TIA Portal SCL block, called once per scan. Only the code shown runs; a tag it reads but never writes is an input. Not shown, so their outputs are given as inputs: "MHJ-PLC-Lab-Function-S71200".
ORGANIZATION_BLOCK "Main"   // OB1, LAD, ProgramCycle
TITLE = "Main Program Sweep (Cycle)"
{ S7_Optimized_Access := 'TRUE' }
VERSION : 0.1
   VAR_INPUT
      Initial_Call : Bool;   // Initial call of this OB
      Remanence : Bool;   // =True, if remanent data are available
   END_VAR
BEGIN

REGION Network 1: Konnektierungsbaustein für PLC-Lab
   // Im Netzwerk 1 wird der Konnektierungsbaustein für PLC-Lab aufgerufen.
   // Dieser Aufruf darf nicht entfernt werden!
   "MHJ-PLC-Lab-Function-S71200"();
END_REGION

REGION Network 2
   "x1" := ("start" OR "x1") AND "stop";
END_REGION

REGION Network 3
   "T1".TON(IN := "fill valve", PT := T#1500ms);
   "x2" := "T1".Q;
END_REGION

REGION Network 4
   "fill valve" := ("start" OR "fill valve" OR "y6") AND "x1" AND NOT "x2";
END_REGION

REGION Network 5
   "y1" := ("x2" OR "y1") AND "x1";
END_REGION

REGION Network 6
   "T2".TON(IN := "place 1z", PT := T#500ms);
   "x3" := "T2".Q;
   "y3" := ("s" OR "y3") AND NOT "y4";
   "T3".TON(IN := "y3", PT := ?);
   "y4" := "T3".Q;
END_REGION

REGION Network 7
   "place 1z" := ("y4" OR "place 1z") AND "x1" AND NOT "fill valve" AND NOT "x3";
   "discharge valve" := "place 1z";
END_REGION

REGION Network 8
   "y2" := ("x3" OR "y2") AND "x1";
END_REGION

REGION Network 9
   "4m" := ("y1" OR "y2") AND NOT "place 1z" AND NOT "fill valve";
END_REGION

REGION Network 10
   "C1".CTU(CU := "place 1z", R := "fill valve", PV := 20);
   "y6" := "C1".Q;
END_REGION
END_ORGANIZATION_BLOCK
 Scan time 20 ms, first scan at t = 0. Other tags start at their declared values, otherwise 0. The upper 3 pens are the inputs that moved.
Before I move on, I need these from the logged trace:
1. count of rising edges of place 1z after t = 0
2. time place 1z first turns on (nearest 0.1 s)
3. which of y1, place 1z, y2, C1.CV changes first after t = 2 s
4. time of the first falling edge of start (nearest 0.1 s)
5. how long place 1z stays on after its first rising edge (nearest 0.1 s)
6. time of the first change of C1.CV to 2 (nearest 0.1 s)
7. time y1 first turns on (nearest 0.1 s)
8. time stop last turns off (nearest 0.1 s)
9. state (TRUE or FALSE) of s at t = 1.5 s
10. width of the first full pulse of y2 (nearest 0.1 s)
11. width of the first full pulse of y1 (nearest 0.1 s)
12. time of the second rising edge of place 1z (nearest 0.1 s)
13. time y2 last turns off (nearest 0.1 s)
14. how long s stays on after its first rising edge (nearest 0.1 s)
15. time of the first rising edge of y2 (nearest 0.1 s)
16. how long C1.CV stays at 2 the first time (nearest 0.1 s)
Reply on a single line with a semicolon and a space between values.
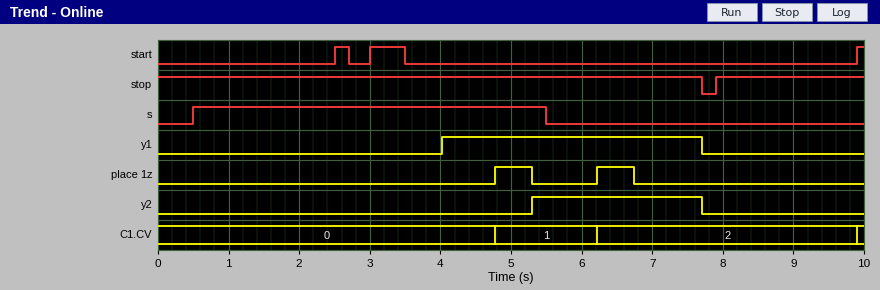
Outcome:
2; 4.8 s; y1; 2.7 s; 0.5 s; 6.2 s; 4.0 s; 7.7 s; TRUE; 2.4 s; 3.7 s; 6.2 s; 7.7 s; 5.0 s; 5.3 s; 3.7 s
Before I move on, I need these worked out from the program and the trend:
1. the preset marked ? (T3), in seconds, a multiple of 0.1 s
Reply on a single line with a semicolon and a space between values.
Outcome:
1.4 s
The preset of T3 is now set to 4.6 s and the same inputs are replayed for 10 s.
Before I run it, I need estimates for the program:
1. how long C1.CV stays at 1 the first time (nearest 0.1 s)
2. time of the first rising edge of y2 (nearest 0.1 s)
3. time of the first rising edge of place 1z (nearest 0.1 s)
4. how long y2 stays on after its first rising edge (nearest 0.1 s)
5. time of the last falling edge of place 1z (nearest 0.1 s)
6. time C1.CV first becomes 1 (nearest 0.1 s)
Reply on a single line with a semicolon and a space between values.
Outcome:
4.8 s; 5.6 s; 5.1 s; 2.1 s; 5.6 s; 5.1 s
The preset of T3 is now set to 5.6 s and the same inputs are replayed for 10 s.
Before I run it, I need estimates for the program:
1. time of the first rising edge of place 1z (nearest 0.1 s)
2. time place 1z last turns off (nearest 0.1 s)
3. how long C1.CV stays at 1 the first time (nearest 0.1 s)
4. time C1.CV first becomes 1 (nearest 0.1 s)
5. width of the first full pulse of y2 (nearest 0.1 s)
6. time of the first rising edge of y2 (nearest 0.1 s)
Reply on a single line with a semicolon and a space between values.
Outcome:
6.1 s; 6.6 s; 3.8 s; 6.1 s; 1.1 s; 6.6 s
